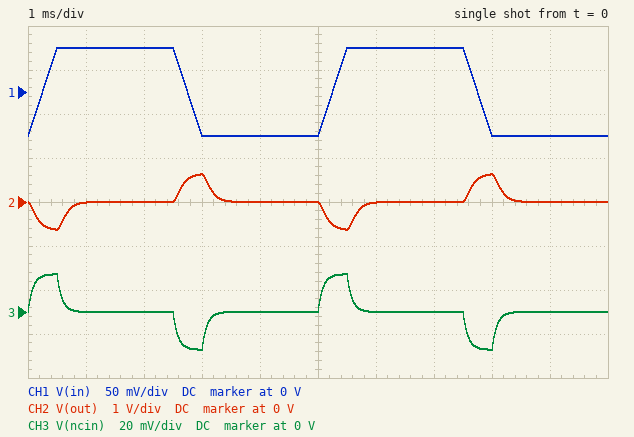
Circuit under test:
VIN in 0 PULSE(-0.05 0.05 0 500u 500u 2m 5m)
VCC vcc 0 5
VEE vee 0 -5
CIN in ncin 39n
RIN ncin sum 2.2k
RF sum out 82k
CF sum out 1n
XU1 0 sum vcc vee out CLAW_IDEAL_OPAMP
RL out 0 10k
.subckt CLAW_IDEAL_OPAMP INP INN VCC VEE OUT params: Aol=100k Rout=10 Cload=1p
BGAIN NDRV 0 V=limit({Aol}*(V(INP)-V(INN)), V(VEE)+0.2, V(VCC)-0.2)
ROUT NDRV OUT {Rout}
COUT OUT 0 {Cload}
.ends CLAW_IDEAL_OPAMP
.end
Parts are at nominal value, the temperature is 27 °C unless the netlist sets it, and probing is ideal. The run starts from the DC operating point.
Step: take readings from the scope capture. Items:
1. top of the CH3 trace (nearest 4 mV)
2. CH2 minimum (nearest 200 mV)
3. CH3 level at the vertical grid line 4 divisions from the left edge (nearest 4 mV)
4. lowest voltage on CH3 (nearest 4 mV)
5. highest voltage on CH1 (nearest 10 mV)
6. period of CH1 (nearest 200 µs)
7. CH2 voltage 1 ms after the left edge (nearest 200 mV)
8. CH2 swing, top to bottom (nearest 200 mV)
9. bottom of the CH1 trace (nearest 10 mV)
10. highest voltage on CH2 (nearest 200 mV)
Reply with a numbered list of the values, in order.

1. 16 mV
2. -600 mV
3. 0 V
4. -16 mV
5. 50 mV
6. 5.0 ms
7. 0 V
8. 1.2 V
9. -50 mV
10. 600 mV
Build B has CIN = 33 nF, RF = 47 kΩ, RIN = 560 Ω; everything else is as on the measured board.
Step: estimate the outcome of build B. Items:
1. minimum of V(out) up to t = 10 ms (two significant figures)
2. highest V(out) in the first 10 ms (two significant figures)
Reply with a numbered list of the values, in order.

1. -310 mV
2. 310 mV
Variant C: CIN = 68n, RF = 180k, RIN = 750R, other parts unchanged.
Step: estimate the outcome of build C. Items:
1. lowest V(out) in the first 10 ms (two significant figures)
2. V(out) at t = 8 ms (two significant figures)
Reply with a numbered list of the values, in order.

1. -2.2 V
2. 2.2 V
